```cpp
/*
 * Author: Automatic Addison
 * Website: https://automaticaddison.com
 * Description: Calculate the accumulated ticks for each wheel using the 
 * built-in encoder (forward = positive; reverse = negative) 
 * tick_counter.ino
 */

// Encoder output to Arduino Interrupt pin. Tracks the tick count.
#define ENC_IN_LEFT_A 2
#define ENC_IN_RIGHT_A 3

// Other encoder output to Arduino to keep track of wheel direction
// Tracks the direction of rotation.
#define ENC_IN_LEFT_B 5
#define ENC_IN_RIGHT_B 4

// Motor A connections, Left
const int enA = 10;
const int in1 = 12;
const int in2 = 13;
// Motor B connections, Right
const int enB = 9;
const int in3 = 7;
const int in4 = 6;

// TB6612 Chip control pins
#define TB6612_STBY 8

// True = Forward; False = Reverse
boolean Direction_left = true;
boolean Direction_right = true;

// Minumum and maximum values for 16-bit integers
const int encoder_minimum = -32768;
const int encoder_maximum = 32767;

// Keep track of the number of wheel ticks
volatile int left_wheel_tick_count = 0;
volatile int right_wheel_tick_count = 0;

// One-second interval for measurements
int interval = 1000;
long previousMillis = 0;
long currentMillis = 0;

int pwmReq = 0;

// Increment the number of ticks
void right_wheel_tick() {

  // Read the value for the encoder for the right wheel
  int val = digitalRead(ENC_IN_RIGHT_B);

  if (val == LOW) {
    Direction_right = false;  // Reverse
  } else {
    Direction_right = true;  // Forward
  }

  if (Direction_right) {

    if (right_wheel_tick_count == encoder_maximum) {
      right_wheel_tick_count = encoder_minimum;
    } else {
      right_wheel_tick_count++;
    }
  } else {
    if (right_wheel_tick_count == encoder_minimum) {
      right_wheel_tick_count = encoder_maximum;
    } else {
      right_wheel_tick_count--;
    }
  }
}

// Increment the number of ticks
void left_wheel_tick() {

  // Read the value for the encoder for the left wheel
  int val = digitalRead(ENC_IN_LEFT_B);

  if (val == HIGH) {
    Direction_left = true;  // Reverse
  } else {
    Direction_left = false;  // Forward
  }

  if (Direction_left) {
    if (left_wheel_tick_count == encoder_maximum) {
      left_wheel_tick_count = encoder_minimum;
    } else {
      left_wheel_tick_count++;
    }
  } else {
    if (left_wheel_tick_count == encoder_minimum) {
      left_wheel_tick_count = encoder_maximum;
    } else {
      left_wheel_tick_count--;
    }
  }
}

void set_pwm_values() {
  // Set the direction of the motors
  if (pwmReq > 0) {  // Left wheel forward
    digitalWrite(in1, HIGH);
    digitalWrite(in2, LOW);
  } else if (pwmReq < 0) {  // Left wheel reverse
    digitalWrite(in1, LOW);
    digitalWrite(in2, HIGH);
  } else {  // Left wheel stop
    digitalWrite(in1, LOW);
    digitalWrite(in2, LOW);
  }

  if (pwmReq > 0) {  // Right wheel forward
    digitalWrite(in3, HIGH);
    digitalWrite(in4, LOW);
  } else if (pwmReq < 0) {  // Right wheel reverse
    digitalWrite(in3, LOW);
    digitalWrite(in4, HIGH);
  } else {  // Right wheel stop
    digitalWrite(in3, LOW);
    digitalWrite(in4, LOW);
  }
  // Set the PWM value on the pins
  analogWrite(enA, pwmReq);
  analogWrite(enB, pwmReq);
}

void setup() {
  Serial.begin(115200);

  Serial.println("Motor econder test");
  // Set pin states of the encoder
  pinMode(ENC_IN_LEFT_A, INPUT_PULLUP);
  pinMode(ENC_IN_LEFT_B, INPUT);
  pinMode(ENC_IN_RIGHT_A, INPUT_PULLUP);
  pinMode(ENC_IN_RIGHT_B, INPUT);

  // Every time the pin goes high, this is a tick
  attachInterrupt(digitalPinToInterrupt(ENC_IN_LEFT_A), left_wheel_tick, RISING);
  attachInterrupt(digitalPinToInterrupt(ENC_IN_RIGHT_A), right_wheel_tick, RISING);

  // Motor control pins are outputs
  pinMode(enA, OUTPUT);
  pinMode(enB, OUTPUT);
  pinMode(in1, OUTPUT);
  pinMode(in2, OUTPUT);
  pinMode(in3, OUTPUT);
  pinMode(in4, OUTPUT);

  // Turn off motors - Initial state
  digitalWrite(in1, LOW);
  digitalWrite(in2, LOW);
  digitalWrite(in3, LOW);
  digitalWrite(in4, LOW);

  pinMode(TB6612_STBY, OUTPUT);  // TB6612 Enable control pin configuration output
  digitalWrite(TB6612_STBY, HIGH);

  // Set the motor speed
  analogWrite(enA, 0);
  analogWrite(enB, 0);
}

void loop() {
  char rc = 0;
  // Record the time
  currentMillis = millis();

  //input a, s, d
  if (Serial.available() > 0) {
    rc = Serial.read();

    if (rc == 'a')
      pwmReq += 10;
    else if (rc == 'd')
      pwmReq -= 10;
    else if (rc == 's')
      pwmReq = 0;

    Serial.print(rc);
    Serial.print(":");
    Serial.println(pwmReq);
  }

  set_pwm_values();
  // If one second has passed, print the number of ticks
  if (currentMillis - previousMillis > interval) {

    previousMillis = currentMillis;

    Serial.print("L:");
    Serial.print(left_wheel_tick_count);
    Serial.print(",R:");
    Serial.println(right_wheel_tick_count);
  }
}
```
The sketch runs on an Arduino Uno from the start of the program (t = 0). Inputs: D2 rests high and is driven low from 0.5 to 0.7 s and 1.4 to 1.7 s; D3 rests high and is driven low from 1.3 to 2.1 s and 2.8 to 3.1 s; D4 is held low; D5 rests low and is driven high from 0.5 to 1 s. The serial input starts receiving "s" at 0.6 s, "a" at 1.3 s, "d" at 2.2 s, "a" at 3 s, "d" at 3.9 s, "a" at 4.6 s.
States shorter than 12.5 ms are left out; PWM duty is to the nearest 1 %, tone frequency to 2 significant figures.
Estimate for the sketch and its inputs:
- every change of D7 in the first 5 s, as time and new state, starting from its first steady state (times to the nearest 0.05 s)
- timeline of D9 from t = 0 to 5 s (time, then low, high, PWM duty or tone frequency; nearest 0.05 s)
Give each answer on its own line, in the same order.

0 s low; 1.3 s high; 2.2 s low; 3 s high; 3.9 s low; 4.6 s high
0 s low; 1.3 s PWM 4 %; 2.2 s low; 3 s PWM 4 %; 3.9 s low; 4.6 s PWM 4 %
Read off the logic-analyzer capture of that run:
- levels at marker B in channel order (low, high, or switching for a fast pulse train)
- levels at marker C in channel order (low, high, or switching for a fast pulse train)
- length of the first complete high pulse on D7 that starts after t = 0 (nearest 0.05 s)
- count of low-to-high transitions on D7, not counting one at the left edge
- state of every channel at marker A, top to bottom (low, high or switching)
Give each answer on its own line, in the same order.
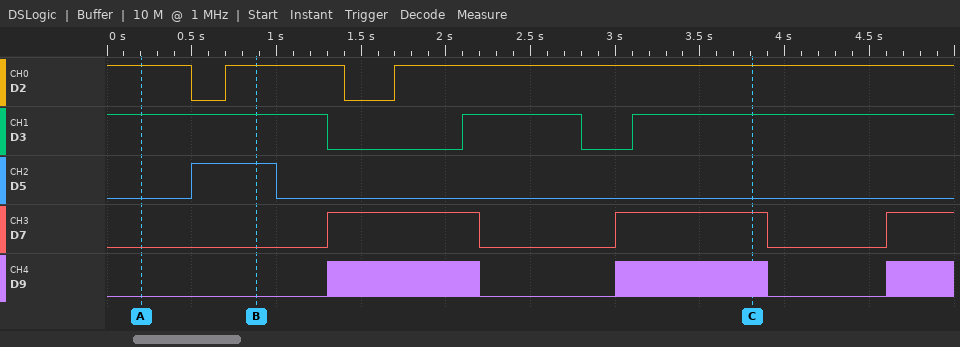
D2 high, D3 high, D5 high, D7 low, D9 low
D2 high, D3 high, D5 low, D7 high, D9 switching
0.90 s
3
D2 high, D3 high, D5 low, D7 low, D9 low
